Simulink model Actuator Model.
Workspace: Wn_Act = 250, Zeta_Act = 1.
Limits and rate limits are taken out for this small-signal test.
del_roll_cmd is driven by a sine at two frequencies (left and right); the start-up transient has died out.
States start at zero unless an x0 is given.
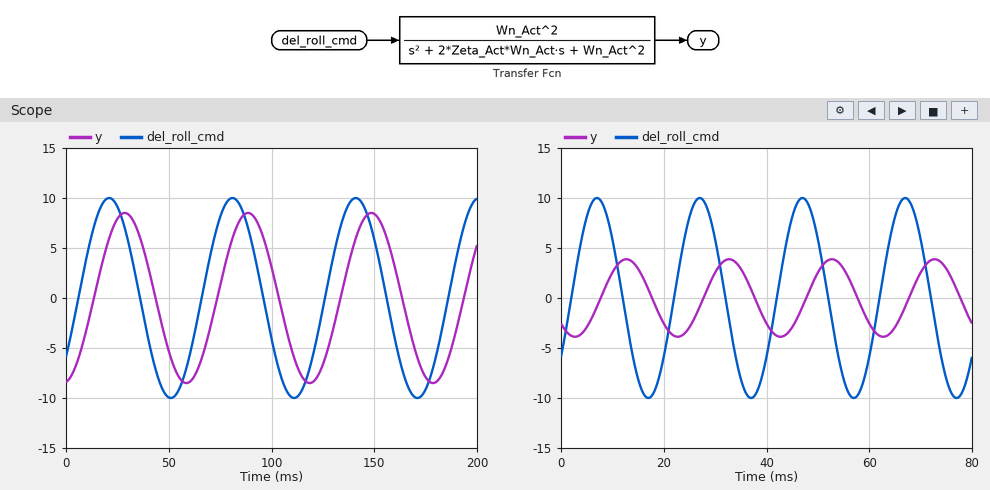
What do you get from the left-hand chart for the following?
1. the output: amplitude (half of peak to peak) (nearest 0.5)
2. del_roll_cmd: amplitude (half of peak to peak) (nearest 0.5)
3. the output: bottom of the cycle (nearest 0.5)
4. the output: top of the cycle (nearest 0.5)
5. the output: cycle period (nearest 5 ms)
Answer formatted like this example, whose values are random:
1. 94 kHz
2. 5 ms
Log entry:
1. 8.5
2. 10.0
3. -8.5
4. 8.5
5. 60 ms
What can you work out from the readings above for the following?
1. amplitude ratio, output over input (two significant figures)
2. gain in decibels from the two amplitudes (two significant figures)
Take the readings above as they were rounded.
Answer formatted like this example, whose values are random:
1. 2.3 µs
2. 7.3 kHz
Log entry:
1. 0.85
2. -1.4 dB
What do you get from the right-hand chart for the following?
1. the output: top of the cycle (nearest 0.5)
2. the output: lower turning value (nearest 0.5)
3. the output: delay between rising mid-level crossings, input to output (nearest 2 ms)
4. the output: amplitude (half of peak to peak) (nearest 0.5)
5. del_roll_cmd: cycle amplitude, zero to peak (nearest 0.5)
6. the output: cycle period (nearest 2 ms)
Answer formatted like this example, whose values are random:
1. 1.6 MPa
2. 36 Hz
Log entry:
1. 4.0
2. -4.0
3. 6 ms
4. 4.0
5. 10.0
6. 20 ms
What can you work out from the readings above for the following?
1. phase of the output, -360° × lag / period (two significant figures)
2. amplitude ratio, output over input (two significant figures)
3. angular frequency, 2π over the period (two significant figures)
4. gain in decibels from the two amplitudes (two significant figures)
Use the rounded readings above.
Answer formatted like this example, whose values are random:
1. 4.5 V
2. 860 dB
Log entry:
1. -110°
2. 0.40
3. 0.31 rad/ms
4. -8.0 dB
